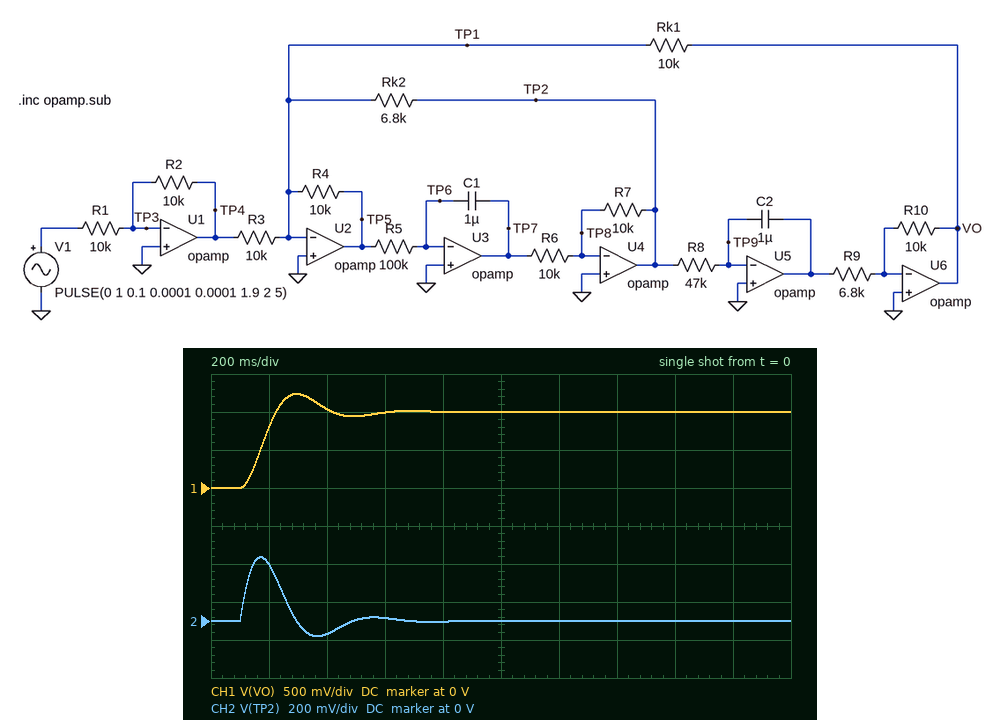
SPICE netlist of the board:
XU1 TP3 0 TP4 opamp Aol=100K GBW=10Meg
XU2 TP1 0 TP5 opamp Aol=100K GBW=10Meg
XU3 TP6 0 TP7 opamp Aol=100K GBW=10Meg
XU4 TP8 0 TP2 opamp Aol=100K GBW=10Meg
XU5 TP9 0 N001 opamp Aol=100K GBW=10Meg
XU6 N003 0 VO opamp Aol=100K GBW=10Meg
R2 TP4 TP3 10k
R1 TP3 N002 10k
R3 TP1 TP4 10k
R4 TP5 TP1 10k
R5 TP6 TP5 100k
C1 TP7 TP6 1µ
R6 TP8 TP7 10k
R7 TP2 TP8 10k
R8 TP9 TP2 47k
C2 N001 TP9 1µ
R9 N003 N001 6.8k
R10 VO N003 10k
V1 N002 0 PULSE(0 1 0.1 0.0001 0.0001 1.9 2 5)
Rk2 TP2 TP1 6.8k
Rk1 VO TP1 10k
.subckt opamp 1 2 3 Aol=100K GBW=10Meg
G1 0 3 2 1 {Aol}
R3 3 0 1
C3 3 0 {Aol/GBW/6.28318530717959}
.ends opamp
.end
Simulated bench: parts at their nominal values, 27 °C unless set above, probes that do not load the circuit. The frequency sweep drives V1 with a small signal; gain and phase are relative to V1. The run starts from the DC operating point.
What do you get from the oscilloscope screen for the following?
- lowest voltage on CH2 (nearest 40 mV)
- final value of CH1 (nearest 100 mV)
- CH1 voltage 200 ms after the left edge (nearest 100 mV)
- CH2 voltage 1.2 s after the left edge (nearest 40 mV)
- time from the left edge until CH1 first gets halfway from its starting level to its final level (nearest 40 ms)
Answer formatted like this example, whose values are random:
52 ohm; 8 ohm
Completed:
-80 mV; 1.0 V; 800 mV; 0 V; 160 ms
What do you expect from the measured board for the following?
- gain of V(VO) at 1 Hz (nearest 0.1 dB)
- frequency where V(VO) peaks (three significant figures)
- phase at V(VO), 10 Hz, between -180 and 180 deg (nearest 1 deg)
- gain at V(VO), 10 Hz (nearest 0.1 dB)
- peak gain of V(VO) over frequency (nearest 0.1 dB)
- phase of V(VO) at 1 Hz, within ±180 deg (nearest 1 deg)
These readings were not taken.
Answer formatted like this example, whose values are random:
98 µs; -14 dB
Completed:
0.7 dB; 2.28 Hz; -166 deg; -21.6 dB; 2.4 dB; -19 deg
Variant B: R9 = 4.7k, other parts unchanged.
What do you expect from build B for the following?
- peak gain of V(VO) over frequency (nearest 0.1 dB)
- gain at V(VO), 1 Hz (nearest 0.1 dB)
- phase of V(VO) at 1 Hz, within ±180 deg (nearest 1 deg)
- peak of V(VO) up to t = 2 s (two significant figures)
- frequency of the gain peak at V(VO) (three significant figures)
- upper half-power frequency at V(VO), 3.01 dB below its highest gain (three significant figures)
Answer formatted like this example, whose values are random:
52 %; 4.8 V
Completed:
3.8 dB; 0.6 dB; -13 deg; 1.3 V; 2.95 Hz; 4.02 Hz
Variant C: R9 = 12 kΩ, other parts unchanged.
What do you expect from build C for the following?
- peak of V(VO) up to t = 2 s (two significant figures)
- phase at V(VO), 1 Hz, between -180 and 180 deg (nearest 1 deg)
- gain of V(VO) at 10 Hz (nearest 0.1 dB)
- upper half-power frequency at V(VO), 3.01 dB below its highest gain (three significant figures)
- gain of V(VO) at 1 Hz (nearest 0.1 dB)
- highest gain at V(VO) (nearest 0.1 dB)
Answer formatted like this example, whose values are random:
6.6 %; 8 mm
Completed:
1.1 V; -34 deg; -26.8 dB; 2.43 Hz; 0.6 dB; 0.7 dB
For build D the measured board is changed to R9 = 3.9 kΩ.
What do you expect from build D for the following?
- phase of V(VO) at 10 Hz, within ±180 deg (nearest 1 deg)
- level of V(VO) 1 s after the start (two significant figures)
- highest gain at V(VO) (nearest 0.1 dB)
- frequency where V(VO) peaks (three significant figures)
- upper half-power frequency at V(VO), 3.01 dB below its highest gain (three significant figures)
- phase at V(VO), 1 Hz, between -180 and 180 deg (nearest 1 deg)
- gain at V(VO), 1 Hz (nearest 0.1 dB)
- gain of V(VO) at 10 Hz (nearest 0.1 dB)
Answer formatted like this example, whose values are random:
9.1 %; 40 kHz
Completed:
-165 deg; 1.0 V; 4.5 dB; 3.33 Hz; 4.40 Hz; -10 deg; 0.5 dB; -16.2 dB
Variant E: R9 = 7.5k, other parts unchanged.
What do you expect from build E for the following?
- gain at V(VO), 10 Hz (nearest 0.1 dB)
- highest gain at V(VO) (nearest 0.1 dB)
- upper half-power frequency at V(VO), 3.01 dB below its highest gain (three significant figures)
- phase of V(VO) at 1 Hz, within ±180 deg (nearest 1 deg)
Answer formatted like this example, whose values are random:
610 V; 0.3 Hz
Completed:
-22.5 dB; 2.1 dB; 3.18 Hz; -21 deg
